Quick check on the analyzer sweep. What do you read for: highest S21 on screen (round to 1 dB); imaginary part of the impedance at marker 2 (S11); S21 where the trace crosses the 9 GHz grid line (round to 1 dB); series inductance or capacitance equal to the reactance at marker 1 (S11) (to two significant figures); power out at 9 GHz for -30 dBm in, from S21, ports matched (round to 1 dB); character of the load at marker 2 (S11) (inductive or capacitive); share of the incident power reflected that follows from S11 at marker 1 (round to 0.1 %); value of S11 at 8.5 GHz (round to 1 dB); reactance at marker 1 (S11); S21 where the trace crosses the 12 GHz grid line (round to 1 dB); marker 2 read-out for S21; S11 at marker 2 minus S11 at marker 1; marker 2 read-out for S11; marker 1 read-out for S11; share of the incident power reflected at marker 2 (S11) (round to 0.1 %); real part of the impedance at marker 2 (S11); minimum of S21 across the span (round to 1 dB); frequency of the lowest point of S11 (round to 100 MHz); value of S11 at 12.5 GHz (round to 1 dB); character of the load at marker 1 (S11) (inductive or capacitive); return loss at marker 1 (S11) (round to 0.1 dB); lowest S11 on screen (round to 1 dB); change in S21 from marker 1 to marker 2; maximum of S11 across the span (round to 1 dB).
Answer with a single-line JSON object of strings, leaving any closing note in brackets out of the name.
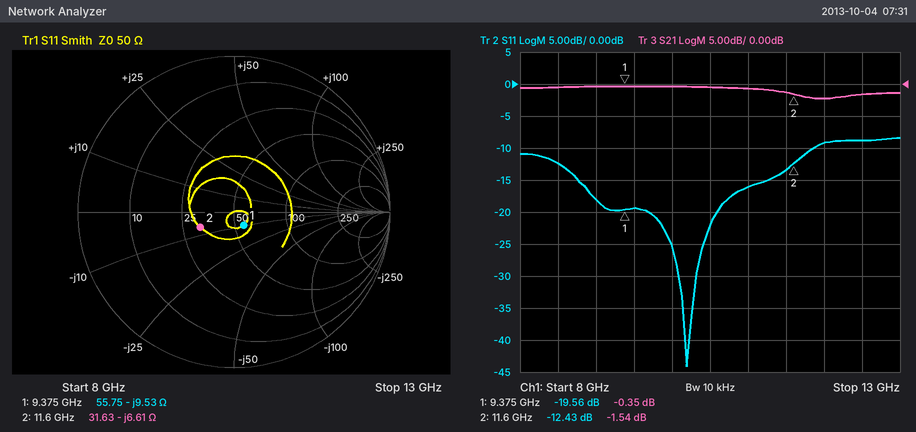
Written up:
{"highest S21 on screen": "0 dB", "imaginary part of the impedance at marker 2": "-6.61 Ω", "S21 where the trace crosses the 9 GHz grid line": "0 dB", "series inductance or capacitance equal to the reactance at marker 1 (S11)": "1.8 pF", "power out at 9 GHz for -30 dBm in, from S21, ports matched": "-30 dBm", "character of the load at marker 2 (S11)": "capacitive", "share of the incident power reflected that follows from S11 at marker 1": "1.1 %", "value of S11 at 8.5 GHz": "-12 dB", "reactance at marker 1": "-9.53 Ω", "S21 where the trace crosses the 12 GHz grid line": "-2 dB", "marker 2 read-out for S21": "-1.54 dB", "S11 at marker 2 minus S11 at marker 1": "7.13 dB", "marker 2 read-out for S11": "-12.43 dB", "marker 1 read-out for S11": "-19.56 dB", "share of the incident power reflected at marker 2 (S11)": "5.7 %", "real part of the impedance at marker 2": "31.63 Ω", "minimum of S21 across the span": "-2 dB", "frequency of the lowest point of S11": "10.2 GHz", "value of S11 at 12.5 GHz": "-9 dB", "character of the load at marker 1 (S11)": "capacitive", "return loss at marker 1 (S11)": "19.6 dB", "lowest S11 on screen": "-44 dB", "change in S21 from marker 1 to marker 2": "-1.19 dB", "maximum of S11 across the span": "-8 dB"}
